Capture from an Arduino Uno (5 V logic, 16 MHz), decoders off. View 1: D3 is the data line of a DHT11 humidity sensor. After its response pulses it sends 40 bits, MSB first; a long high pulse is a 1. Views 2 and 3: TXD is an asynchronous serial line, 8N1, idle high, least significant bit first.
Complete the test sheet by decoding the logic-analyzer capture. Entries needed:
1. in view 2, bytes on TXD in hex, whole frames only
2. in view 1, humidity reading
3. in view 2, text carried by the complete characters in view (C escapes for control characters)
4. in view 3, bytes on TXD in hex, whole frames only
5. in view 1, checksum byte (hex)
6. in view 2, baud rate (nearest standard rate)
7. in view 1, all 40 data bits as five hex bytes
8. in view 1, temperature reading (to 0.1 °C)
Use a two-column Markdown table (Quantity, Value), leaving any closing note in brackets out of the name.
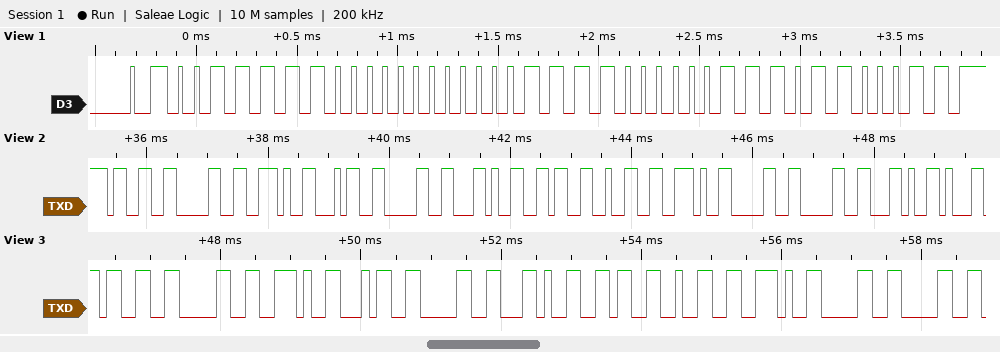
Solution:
| Quantity | Value |
|---|---|
| in view 2, bytes on TXD in hex, whole frames only | 0x33 0x30 0x2E 0x34 0x30 0x2C 0x36 0x32 0x2E 0x30 0x30 0x2C |
| in view 1, humidity reading | 62 % |
| in view 2, text carried by the complete characters in view | "30.40,62.00," |
| in view 3, bytes on TXD in hex, whole frames only | 33 30 2E 34 30 2C 36 32 2E 30 30 |
| in view 1, checksum byte | 0x63 |
| in view 2, baud rate | 9600 baud |
| in view 1, all 40 data bits as five hex bytes | 3E 00 1E 07 63 |
| in view 1, temperature reading | 30.7 °C |
